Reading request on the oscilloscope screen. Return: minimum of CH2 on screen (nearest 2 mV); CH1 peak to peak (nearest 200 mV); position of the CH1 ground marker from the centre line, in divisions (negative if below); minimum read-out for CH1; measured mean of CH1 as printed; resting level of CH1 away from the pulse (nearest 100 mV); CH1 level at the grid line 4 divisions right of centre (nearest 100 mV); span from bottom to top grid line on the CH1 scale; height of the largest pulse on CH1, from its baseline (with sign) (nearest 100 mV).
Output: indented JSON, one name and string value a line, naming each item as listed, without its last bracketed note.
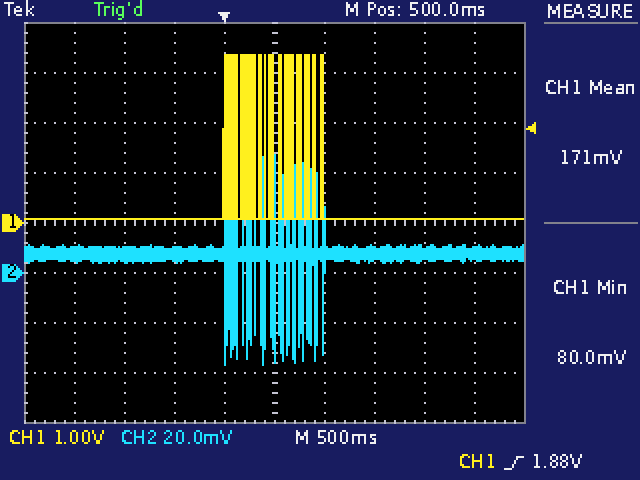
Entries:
{
  "minimum of CH2 on screen": "-36 mV",
  "CH1 peak to peak": "3.2 V",
  "position of the CH1 ground marker from the centre line, in divisions": "0.0 div",
  "minimum read-out for CH1": "80.0 mV",
  "measured mean of CH1 as printed": "171 mV",
  "resting level of CH1 away from the pulse": "100 mV",
  "CH1 level at the grid line 4 divisions right of centre": "100 mV",
  "span from bottom to top grid line on the CH1 scale": "8 V",
  "height of the largest pulse on CH1, from its baseline (with sign)": "+3.3 V"
}
